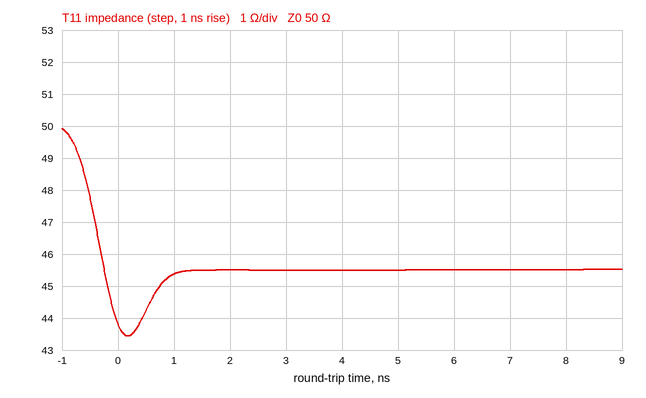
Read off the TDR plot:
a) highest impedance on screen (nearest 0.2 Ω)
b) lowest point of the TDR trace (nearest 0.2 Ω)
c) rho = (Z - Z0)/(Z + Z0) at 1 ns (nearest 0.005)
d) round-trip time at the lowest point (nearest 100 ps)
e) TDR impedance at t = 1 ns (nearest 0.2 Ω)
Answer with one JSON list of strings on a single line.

["50.0 Ω", "43.4 Ω", "-0.050", "200 ps", "45.4 Ω"]
